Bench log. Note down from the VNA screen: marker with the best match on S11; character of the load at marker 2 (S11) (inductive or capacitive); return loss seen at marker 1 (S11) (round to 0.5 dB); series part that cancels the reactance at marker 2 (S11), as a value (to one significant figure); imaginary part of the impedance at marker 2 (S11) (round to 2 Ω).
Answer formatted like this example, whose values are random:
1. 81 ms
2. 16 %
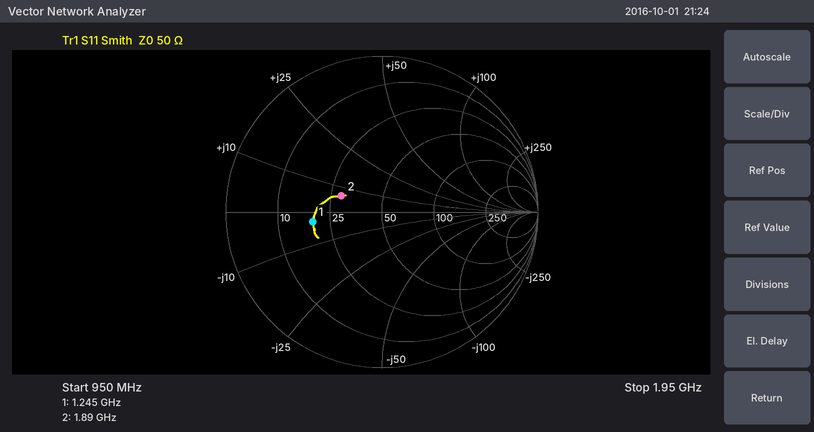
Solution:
1. marker 2
2. inductive
3. 7.0 dB
4. 10 pF
5. +6 Ω
